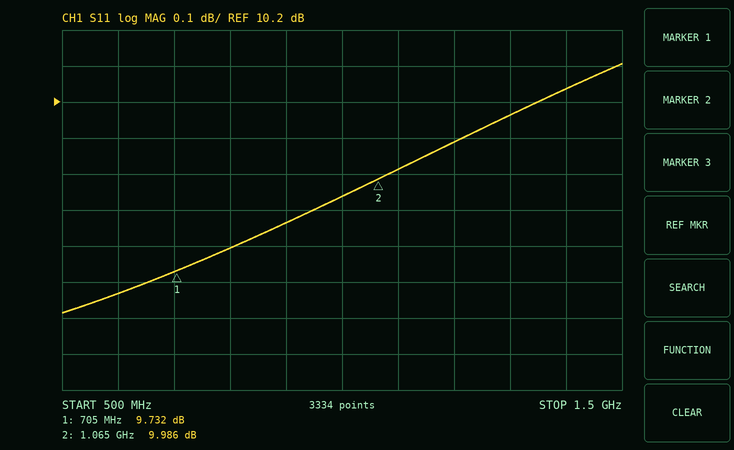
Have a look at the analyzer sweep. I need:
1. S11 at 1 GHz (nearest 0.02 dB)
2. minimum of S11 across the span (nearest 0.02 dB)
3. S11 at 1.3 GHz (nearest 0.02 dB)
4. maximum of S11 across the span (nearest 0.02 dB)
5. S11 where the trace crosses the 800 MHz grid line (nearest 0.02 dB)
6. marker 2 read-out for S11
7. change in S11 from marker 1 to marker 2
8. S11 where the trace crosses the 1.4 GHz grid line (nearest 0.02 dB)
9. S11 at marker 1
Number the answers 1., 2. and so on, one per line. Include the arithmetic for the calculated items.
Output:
1. 9.94 dB
2. 9.62 dB
3. 10.16 dB
4. 10.30 dB
5. 9.80 dB
6. 9.986 dB
7. 9.986 − (9.732) = 0.254 dB
8. 10.24 dB
9. 9.732 dB
